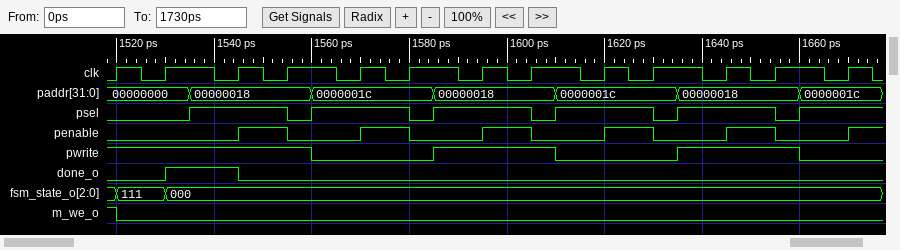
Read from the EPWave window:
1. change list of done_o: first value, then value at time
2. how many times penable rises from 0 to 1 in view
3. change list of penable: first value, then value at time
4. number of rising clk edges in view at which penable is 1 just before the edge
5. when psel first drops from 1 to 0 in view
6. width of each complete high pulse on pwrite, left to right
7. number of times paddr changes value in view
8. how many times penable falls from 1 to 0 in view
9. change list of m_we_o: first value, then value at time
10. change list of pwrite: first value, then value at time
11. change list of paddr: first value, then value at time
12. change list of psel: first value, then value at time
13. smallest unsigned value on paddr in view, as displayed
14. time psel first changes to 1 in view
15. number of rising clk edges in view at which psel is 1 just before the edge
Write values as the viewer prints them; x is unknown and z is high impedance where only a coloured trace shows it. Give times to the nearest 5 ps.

0, 1 at 1530 ps, 0 at 1545 ps
6
0, 1 at 1545 ps, 0 at 1555 ps, 1 at 1570 ps, 0 at 1580 ps, 1 at 1595 ps, 0 at 1605 ps, 1 at 1620 ps, 0 at 1630 ps, 1 at 1645 ps, 0 at 1655 ps, 1 at 1670 ps
5
1555 ps
25 ps, 25 ps
6
5
1, 0 at 1520 ps
1, 0 at 1560 ps, 1 at 1585 ps, 0 at 1610 ps, 1 at 1635 ps, 0 at 1660 ps
00000000, 00000018 at 1535 ps, 0000001c at 1560 ps, 00000018 at 1585 ps, 0000001c at 1610 ps, 00000018 at 1635 ps, 0000001c at 1660 ps
0, 1 at 1535 ps, 0 at 1555 ps, 1 at 1560 ps, 0 at 1580 ps, 1 at 1585 ps, 0 at 1605 ps, 1 at 1610 ps, 0 at 1630 ps, 1 at 1635 ps, 0 at 1655 ps, 1 at 1660 ps
00000000
1535 ps
11
